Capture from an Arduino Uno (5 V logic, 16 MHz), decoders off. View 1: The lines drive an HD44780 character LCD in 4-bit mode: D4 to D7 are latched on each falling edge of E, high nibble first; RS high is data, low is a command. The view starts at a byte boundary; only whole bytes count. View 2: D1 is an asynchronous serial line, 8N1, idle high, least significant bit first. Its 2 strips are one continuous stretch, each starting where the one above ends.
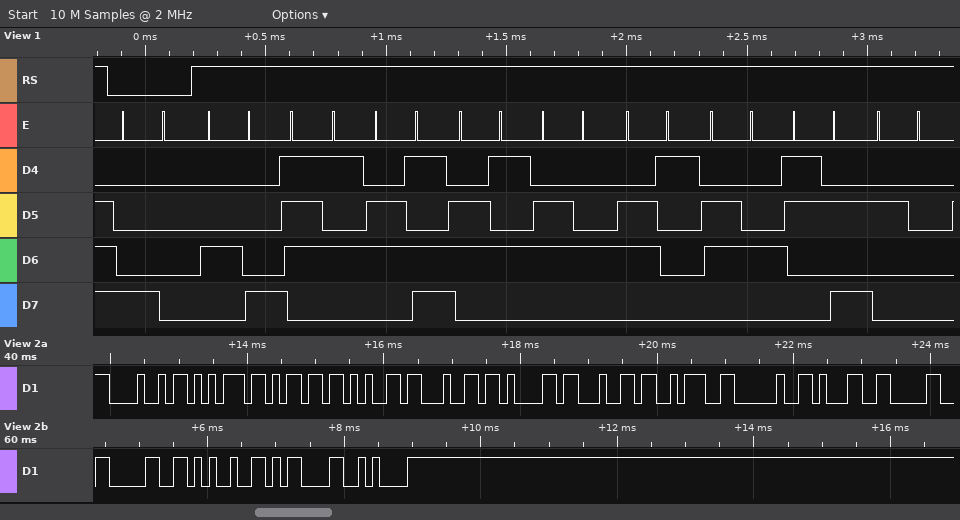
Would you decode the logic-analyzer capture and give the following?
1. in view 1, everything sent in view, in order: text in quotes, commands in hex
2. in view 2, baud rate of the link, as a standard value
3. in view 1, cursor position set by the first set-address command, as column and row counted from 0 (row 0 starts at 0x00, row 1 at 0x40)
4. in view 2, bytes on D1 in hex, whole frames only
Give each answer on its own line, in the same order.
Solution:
0x80 "Humedad: "
9600 baud
column 0, row 0
48 75 6D 65 64 61 64 3A 20 31 30 30 25 0D 0A
